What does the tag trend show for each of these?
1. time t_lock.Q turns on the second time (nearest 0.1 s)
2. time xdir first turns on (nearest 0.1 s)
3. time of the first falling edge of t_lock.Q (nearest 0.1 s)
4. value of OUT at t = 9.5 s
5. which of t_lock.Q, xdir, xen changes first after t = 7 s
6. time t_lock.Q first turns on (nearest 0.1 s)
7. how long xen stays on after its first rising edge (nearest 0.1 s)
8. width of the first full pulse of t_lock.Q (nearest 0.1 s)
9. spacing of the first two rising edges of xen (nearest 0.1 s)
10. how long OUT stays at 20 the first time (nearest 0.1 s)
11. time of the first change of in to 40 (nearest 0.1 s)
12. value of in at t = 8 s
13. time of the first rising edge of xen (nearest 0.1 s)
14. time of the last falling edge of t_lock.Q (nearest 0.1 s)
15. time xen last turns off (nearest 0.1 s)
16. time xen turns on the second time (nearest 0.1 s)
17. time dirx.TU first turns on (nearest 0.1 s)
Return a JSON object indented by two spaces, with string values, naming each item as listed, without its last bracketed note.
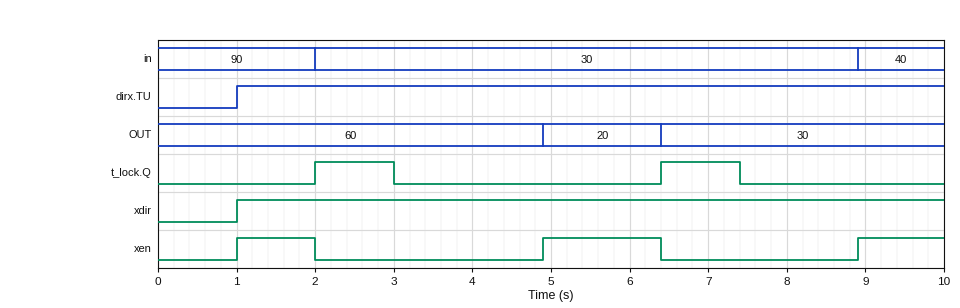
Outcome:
{
  "time t_lock.Q turns on the second time": "6.4 s",
  "time xdir first turns on": "1.0 s",
  "time of the first falling edge of t_lock.Q": "3.0 s",
  "value of OUT at t = 9.5 s": "30",
  "which of t_lock.Q, xdir, xen changes first after t = 7 s": "t_lock.Q",
  "time t_lock.Q first turns on": "2.0 s",
  "how long xen stays on after its first rising edge": "1.0 s",
  "width of the first full pulse of t_lock.Q": "1.0 s",
  "spacing of the first two rising edges of xen": "3.9 s",
  "how long OUT stays at 20 the first time": "1.5 s",
  "time of the first change of in to 40": "8.9 s",
  "value of in at t = 8 s": "30",
  "time of the first rising edge of xen": "1.0 s",
  "time of the last falling edge of t_lock.Q": "7.4 s",
  "time xen last turns off": "6.4 s",
  "time xen turns on the second time": "4.9 s",
  "time dirx.TU first turns on": "1.0 s"
}
